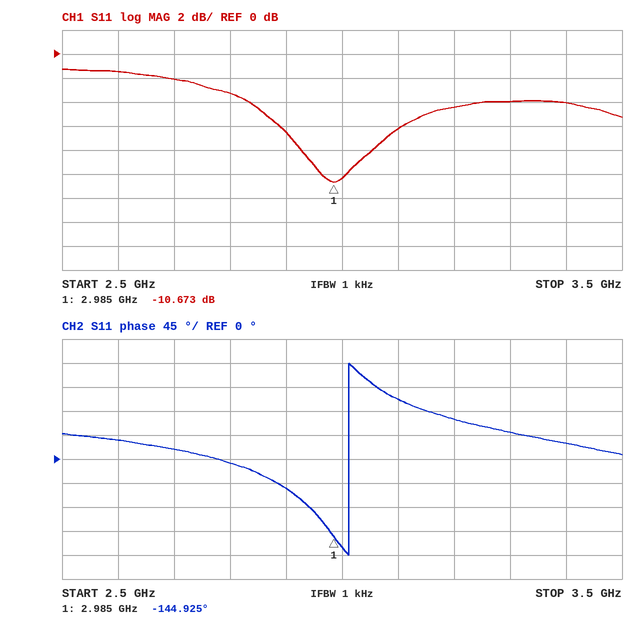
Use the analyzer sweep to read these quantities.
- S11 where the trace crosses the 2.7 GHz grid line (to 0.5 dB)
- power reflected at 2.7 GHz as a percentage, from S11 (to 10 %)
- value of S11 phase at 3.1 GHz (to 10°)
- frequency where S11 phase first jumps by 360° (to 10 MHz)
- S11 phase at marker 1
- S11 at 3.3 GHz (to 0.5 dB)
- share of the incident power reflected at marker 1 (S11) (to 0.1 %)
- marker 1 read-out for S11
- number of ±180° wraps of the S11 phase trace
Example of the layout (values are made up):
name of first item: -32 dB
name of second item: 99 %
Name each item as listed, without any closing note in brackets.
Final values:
S11 where the trace crosses the 2.7 GHz grid line: -2.0 dB
power reflected at 2.7 GHz as a percentage, from S11: 60 %
value of S11 phase at 3.1 GHz: 110°
frequency where S11 phase first jumps by 360°: 3.01 GHz
S11 phase at marker 1: -144.925°
S11 at 3.3 GHz: -4.0 dB
share of the incident power reflected at marker 1 (S11): 8.6 %
marker 1 read-out for S11: -10.673 dB
number of ±180° wraps of the S11 phase trace: 1
